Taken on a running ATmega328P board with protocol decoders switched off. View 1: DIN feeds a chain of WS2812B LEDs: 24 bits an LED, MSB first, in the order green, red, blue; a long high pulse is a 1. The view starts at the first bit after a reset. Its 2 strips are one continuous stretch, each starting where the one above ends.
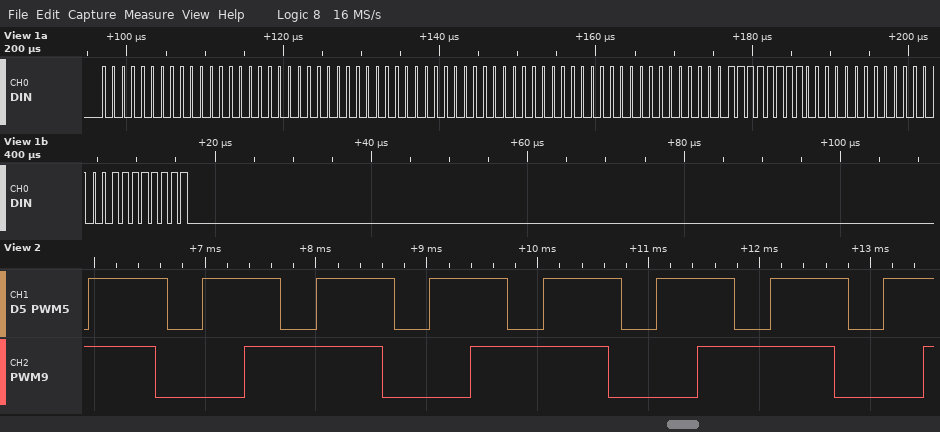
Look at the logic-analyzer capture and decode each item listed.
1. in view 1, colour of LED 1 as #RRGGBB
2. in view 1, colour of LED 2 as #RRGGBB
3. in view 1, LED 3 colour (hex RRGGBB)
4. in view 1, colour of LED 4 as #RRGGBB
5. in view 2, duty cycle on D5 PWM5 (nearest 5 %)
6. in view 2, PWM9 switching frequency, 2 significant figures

#000000
#000000
#0000FF
#0000FF
70 %
490 Hz
